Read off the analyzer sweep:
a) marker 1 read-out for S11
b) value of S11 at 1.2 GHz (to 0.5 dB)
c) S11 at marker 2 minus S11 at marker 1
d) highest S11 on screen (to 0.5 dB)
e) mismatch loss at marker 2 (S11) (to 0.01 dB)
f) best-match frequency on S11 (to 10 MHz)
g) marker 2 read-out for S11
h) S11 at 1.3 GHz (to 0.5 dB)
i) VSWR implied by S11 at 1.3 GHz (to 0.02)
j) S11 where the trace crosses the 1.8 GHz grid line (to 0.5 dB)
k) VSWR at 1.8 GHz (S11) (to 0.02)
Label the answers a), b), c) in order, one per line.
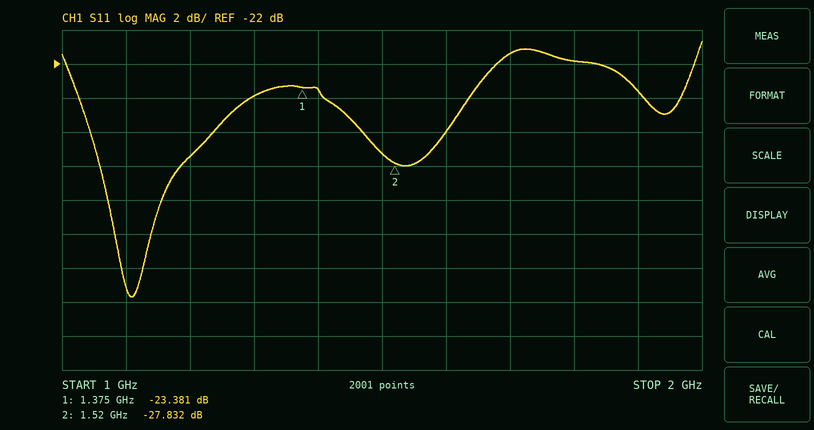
a) -23.381 dB
b) -27.5 dB
c) -4.451 dB
d) -20.5 dB
e) 0.01 dB
f) 1.11 GHz
g) -27.832 dB
h) -24.0 dB
i) 1.14
j) -22.0 dB
k) 1.18
